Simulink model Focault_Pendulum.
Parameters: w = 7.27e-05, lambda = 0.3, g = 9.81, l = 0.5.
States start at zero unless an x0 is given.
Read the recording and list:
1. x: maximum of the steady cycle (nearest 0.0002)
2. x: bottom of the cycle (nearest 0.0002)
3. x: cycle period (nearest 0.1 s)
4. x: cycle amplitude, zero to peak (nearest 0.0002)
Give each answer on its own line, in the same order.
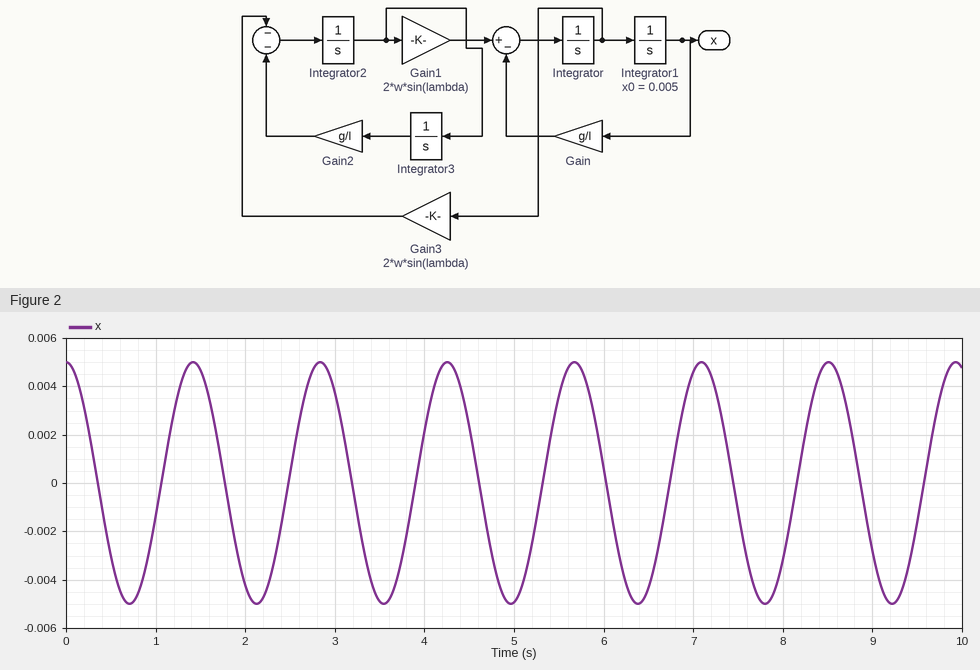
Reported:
0.0050
-0.0050
1.4 s
0.0050
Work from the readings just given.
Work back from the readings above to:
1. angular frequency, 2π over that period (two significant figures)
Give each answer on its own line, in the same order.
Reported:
4.5 rad/s
